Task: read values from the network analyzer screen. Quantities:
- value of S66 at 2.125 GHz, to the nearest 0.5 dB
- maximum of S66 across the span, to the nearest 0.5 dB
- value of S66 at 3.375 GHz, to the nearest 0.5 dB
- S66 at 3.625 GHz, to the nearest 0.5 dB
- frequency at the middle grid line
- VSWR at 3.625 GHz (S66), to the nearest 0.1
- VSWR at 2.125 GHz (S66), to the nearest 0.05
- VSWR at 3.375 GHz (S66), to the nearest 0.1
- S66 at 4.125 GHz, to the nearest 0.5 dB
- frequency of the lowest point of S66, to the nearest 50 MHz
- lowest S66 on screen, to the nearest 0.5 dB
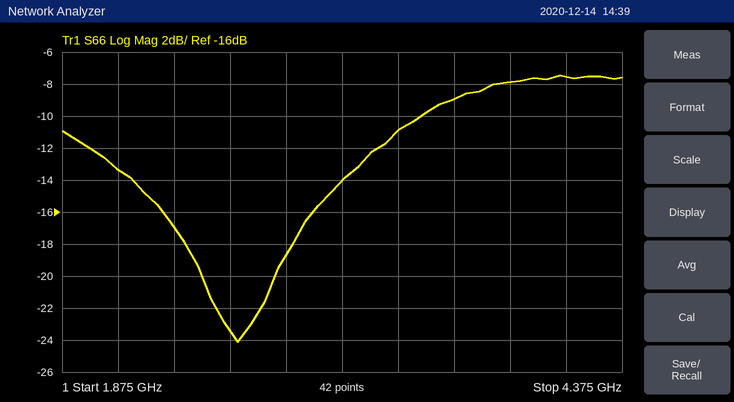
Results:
-13.5 dB
-7.5 dB
-11.0 dB
-9.0 dB
3.125 GHz
2.1
1.55
1.8
-7.5 dB
2.65 GHz
-24.0 dB
